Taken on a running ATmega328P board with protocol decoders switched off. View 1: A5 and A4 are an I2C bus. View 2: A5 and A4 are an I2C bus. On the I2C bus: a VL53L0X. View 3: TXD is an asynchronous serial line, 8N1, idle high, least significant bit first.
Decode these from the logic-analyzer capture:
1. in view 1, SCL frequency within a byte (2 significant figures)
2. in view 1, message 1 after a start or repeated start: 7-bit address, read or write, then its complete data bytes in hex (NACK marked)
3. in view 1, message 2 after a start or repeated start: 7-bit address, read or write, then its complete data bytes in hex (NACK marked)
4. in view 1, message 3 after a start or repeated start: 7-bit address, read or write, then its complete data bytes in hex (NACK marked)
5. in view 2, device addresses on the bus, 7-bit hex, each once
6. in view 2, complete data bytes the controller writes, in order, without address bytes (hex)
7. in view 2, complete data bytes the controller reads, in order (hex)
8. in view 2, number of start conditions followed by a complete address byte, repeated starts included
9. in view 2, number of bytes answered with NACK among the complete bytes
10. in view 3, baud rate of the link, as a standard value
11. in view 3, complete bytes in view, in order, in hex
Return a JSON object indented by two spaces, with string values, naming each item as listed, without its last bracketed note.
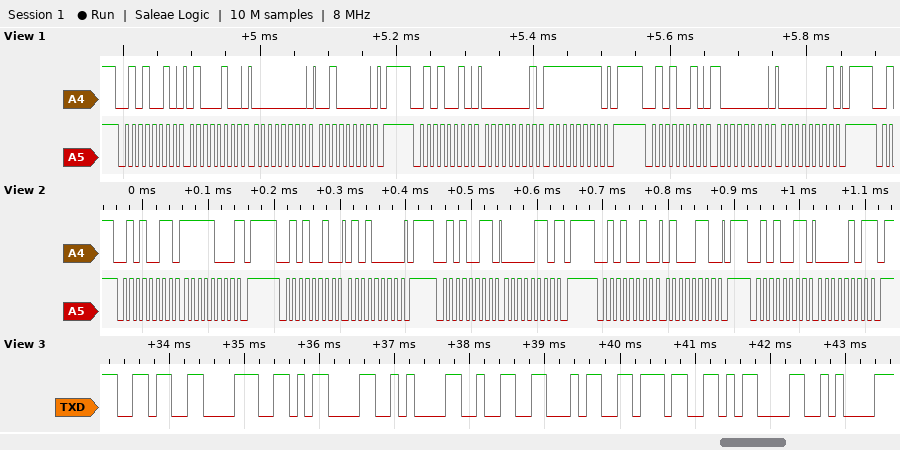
{
  "in view 1, SCL frequency within a byte": "100 kHz",
  "in view 1, message 1 after a start or repeated start: 7-bit address, read or write, then its complete data bytes in hex": "0x29 write: 44 00 20",
  "in view 1, message 2 after a start or repeated start: 7-bit address, read or write, then its complete data bytes in hex": "0x29 write: 01 FF",
  "in view 1, message 3 after a start or repeated start: 7-bit address, read or write, then its complete data bytes in hex": "0x29 write: 80 01",
  "in view 2, device addresses on the bus, 7-bit hex, each once": "0x29",
  "in view 2, complete data bytes the controller writes, in order, without address bytes": "50 46",
  "in view 2, complete data bytes the controller reads, in order": "F8 06 05",
  "in view 2, number of start conditions followed by a complete address byte, repeated starts included": "5",
  "in view 2, number of bytes answered with NACK among the complete bytes": "3",
  "in view 3, baud rate of the link, as a standard value": "9600 baud",
  "in view 3, complete bytes in view, in order, in hex": "0x36 0x38 0x0D 0x0A 0x32 0x34 0x37 0x0D 0x0A"
}
